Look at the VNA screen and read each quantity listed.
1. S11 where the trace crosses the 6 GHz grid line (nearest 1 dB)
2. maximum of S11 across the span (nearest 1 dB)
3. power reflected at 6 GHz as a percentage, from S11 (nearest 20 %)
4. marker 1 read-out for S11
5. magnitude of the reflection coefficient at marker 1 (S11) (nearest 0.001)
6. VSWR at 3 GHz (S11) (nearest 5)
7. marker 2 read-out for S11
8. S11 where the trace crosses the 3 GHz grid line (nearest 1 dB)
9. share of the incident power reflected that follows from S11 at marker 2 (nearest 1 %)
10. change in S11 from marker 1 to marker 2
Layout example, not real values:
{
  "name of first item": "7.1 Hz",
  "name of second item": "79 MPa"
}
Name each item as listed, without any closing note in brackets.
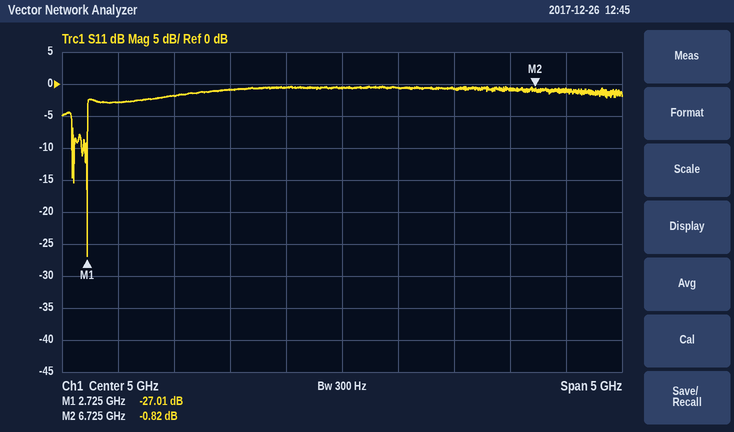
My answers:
{
  "S11 where the trace crosses the 6 GHz grid line": "-1 dB",
  "maximum of S11 across the span": "0 dB",
  "power reflected at 6 GHz as a percentage, from S11": "80 %",
  "marker 1 read-out for S11": "-27.01 dB",
  "magnitude of the reflection coefficient at marker 1 (S11)": "0.045",
  "VSWR at 3 GHz (S11)": "5",
  "marker 2 read-out for S11": "-0.82 dB",
  "S11 where the trace crosses the 3 GHz grid line": "-3 dB",
  "share of the incident power reflected that follows from S11 at marker 2": "83 %",
  "change in S11 from marker 1 to marker 2": "26.19 dB"
}
